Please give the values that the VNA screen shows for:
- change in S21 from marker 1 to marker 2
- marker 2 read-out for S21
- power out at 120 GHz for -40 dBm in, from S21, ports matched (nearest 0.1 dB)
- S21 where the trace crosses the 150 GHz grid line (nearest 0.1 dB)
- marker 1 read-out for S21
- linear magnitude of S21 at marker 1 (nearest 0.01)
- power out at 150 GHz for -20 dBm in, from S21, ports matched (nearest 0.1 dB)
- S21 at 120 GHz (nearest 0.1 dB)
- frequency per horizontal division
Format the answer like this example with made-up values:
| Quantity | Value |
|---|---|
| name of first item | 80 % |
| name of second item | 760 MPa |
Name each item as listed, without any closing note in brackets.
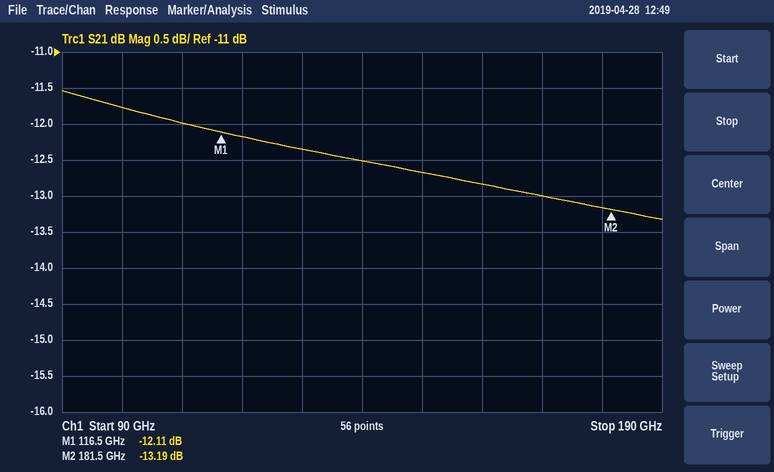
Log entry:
| Quantity | Value |
|---|---|
| change in S21 from marker 1 to marker 2 | -1.08 dB |
| marker 2 read-out for S21 | -13.19 dB |
| power out at 120 GHz for -40 dBm in, from S21, ports matched | -52.2 dBm |
| S21 where the trace crosses the 150 GHz grid line | -12.7 dB |
| marker 1 read-out for S21 | -12.11 dB |
| linear magnitude of S21 at marker 1 | 0.25 |
| power out at 150 GHz for -20 dBm in, from S21, ports matched | -32.7 dBm |
| S21 at 120 GHz | -12.2 dB |
| frequency per horizontal division | 10 GHz |
